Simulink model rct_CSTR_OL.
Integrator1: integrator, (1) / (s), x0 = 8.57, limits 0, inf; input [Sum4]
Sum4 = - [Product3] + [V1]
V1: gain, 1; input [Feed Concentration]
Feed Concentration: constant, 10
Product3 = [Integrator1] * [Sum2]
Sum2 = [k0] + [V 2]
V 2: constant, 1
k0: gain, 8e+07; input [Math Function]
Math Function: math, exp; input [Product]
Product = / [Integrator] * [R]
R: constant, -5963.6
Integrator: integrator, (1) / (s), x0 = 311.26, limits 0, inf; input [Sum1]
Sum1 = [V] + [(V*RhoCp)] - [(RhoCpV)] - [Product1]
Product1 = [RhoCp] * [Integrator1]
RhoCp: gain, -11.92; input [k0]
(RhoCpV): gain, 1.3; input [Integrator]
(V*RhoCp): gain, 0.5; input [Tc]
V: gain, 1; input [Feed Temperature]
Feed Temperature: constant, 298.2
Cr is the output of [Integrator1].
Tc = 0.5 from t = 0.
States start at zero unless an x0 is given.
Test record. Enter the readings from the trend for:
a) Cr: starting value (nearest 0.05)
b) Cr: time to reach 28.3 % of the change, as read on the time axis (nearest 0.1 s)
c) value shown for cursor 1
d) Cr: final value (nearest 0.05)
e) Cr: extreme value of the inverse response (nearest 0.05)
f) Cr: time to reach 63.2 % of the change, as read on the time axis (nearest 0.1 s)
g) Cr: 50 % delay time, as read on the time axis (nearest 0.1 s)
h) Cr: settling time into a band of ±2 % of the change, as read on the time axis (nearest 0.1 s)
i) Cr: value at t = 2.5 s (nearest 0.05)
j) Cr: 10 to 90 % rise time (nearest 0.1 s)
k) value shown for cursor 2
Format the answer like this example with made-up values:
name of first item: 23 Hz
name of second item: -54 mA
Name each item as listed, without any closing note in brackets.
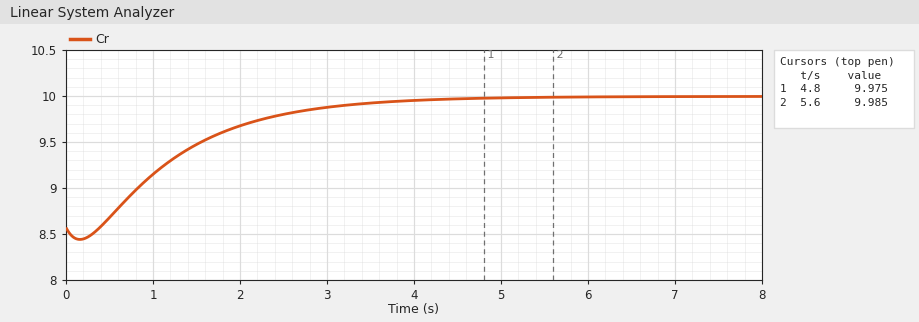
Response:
Cr: starting value: 8.55
Cr: time to reach 28.3 % of the change, as read on the time axis: 0.8 s
value shown for cursor 1: 9.975
Cr: final value: 10.00
Cr: extreme value of the inverse response: 8.45
Cr: time to reach 63.2 % of the change, as read on the time axis: 1.5 s
Cr: 50 % delay time, as read on the time axis: 1.2 s
Cr: settling time into a band of ±2 % of the change, as read on the time axis: 4.4 s
Cr: value at t = 2.5 s: 9.80
Cr: 10 to 90 % rise time: 2.3 s
value shown for cursor 2: 9.985
